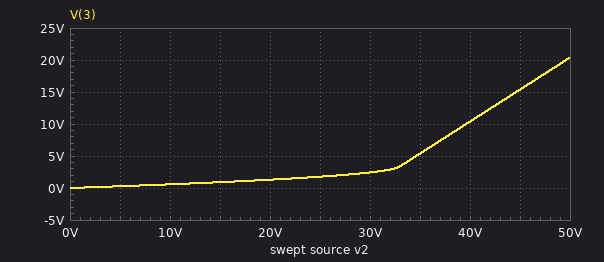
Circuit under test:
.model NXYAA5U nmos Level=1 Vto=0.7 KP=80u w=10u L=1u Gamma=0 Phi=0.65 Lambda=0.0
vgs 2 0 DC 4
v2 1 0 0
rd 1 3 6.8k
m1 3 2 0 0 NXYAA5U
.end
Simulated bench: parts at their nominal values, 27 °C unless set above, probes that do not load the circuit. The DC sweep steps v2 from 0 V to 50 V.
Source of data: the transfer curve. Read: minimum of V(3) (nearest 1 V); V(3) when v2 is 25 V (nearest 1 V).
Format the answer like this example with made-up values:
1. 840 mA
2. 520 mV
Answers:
1. 0 V
2. 2 V
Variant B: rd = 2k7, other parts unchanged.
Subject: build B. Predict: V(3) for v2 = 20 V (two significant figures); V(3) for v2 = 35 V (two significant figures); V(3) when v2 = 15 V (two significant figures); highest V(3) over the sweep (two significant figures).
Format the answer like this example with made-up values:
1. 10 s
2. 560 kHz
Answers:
1. 8.2 V
2. 23 V
3. 3.2 V
4. 38 V
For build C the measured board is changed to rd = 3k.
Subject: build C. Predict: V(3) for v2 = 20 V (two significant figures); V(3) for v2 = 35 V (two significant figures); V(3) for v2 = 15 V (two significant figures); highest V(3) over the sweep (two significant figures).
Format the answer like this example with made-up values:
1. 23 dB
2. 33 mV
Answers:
1. 6.9 V
2. 22 V
3. 2.6 V
4. 37 V
